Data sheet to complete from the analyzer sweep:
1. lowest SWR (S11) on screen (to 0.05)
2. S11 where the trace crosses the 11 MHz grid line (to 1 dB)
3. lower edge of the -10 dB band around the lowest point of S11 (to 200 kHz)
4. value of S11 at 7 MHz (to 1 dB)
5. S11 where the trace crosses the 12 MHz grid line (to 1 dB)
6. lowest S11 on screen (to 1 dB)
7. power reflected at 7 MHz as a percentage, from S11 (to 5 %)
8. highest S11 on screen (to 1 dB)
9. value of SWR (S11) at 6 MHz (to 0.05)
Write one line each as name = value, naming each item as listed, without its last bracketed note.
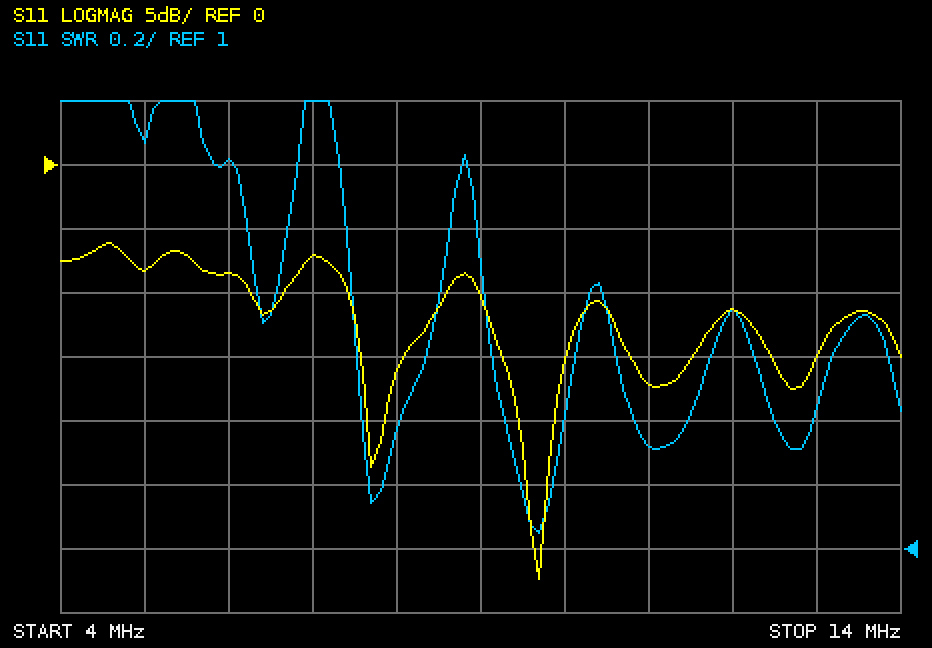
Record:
lowest SWR (S11) on screen = 1.05
S11 where the trace crosses the 11 MHz grid line = -17 dB
lower edge of the -10 dB band around the lowest point of S11 = 9.0 MHz
value of S11 at 7 MHz = -7 dB
S11 where the trace crosses the 12 MHz grid line = -11 dB
lowest S11 on screen = -32 dB
power reflected at 7 MHz as a percentage, from S11 = 20 %
highest S11 on screen = -6 dB
value of SWR (S11) at 6 MHz = 2.20
